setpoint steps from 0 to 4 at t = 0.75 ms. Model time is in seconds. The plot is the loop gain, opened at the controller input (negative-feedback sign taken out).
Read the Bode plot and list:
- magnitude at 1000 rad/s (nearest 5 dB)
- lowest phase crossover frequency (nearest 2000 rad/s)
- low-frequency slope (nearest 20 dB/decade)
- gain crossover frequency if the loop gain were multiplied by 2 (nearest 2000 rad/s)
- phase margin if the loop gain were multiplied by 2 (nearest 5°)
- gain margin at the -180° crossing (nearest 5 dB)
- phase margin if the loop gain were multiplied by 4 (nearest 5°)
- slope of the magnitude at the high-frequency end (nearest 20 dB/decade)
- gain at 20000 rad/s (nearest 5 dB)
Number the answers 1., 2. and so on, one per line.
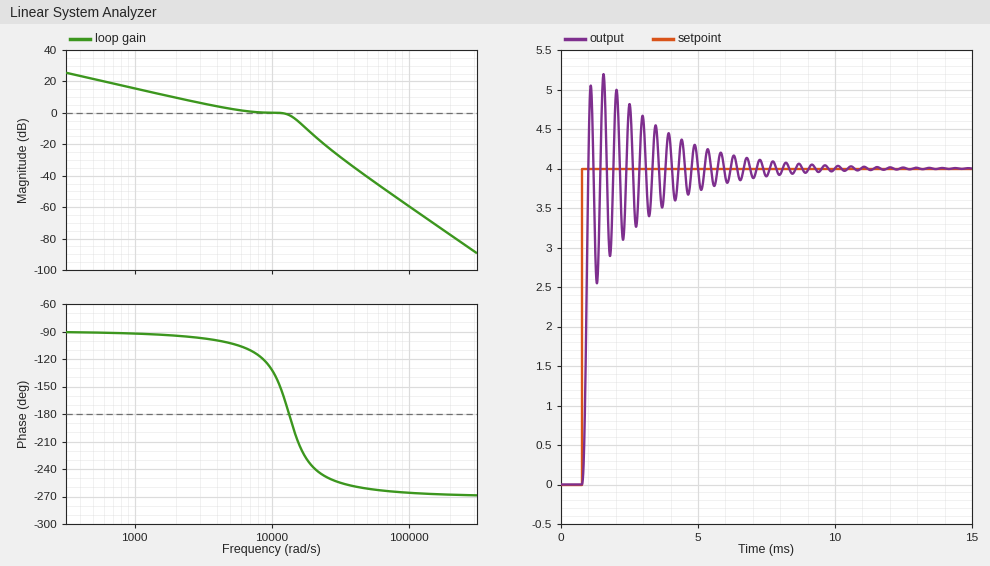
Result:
1. 15 dB
2. 14000 rad/s
3. -20 dB/decade
4. 16000 rad/s
5. -35°
6. 0 dB
7. -55°
8. -60 dB/decade
9. -15 dB
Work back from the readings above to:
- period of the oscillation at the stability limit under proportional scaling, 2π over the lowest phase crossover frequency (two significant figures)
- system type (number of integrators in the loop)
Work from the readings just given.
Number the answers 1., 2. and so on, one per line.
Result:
1. 0.00045 s
2. 1
